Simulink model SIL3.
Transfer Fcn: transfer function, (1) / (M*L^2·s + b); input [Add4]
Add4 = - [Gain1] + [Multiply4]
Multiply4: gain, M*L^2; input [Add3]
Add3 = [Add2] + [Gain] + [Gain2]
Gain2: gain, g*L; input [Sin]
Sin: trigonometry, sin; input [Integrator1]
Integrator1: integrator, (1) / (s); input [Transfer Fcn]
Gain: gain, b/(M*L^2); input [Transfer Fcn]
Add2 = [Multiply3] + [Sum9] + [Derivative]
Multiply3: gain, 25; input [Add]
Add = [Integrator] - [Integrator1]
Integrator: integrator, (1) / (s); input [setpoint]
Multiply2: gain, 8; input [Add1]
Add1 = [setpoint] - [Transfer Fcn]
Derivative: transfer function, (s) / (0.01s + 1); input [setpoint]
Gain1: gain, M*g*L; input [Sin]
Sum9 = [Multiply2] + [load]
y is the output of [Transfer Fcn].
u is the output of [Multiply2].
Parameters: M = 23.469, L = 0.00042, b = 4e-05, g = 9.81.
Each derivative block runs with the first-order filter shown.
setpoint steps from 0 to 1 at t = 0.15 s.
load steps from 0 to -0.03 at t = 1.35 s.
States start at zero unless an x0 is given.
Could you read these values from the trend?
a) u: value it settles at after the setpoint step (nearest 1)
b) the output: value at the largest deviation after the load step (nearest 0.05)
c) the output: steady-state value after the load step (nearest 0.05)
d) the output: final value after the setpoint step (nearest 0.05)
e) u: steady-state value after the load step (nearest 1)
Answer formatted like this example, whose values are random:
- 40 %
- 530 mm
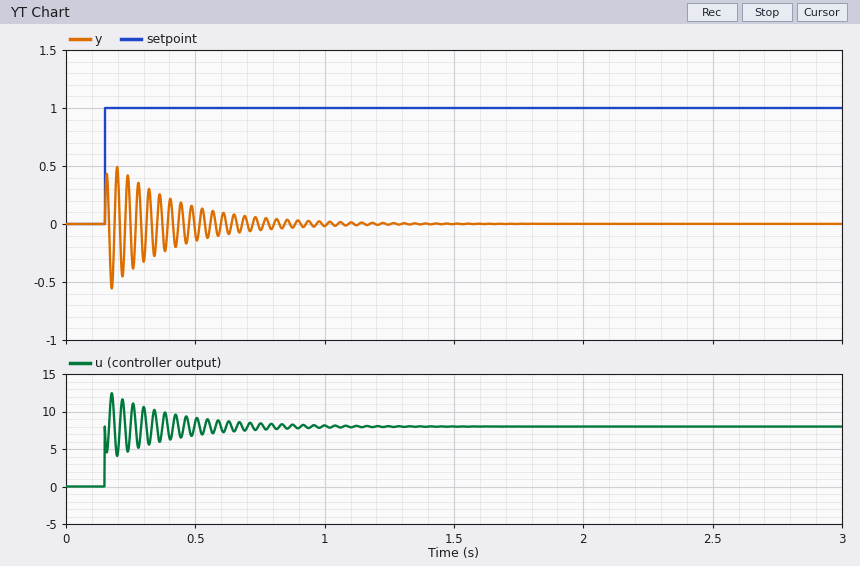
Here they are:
- 8
- 0.00
- 0.00
- 0.00
- 8
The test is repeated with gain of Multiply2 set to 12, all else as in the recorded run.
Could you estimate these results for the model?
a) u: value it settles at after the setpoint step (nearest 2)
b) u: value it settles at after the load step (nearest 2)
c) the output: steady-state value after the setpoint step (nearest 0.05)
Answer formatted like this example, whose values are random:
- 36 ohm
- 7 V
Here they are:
- 12
- 12
- 0.00
